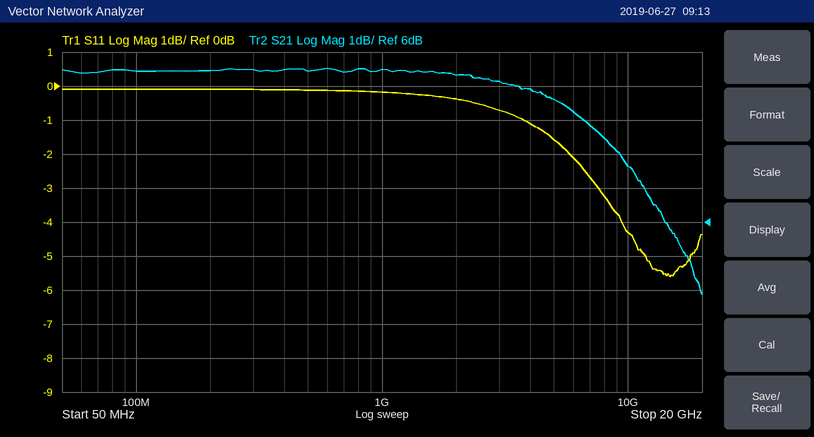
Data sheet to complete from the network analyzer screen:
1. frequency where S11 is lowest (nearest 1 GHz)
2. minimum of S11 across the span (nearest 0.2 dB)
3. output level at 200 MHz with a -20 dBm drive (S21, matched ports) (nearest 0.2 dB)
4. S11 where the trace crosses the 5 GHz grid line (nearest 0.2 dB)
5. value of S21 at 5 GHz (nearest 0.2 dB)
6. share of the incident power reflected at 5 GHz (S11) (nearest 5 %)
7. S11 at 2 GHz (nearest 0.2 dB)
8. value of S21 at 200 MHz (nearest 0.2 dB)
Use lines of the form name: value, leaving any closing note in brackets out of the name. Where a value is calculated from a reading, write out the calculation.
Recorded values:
frequency where S11 is lowest: 15 GHz
minimum of S11 across the span: -5.6 dB
output level at 200 MHz with a -20 dBm drive (S21, matched ports): -20 dBm + (10.4 dB) = -9.6 dBm
S11 where the trace crosses the 5 GHz grid line: -1.6 dB
value of S21 at 5 GHz: 9.6 dB
share of the incident power reflected at 5 GHz (S11): 10^(-1.6/10) ≈ 69.2 %, so 70 % to the nearest 5 %
S11 at 2 GHz: -0.4 dB
value of S21 at 200 MHz: 10.4 dB
